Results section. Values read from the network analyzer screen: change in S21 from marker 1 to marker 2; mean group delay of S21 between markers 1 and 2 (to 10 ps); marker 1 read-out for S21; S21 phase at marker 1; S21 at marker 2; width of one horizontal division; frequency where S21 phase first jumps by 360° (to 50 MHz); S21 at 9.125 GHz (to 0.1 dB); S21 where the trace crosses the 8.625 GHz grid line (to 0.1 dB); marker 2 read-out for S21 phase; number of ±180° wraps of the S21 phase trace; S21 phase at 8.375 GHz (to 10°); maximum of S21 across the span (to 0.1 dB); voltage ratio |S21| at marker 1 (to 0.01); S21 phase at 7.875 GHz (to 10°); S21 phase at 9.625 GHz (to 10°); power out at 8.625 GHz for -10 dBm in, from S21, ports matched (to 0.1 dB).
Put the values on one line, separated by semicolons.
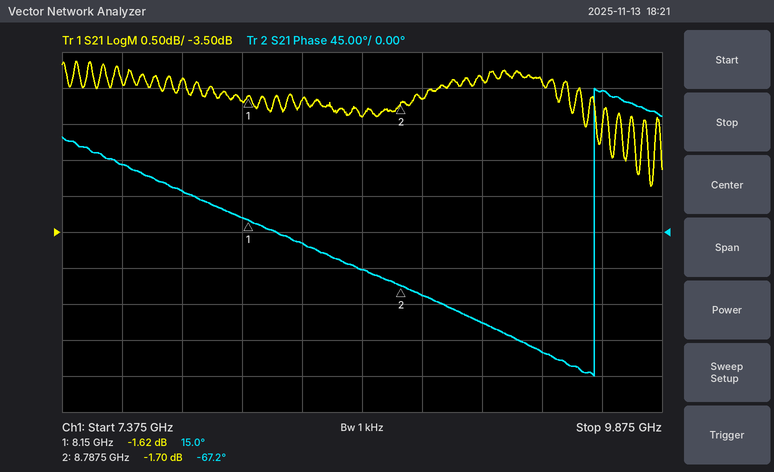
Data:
-0.08 dB; 360 ps; -1.62 dB; 15.0°; -1.70 dB; 250 MHz; 9.60 GHz; -1.4 dB; -1.9 dB; -67.2°; 1; -10°; -1.1 dB; 0.83; 50°; 180°; -11.9 dBm
